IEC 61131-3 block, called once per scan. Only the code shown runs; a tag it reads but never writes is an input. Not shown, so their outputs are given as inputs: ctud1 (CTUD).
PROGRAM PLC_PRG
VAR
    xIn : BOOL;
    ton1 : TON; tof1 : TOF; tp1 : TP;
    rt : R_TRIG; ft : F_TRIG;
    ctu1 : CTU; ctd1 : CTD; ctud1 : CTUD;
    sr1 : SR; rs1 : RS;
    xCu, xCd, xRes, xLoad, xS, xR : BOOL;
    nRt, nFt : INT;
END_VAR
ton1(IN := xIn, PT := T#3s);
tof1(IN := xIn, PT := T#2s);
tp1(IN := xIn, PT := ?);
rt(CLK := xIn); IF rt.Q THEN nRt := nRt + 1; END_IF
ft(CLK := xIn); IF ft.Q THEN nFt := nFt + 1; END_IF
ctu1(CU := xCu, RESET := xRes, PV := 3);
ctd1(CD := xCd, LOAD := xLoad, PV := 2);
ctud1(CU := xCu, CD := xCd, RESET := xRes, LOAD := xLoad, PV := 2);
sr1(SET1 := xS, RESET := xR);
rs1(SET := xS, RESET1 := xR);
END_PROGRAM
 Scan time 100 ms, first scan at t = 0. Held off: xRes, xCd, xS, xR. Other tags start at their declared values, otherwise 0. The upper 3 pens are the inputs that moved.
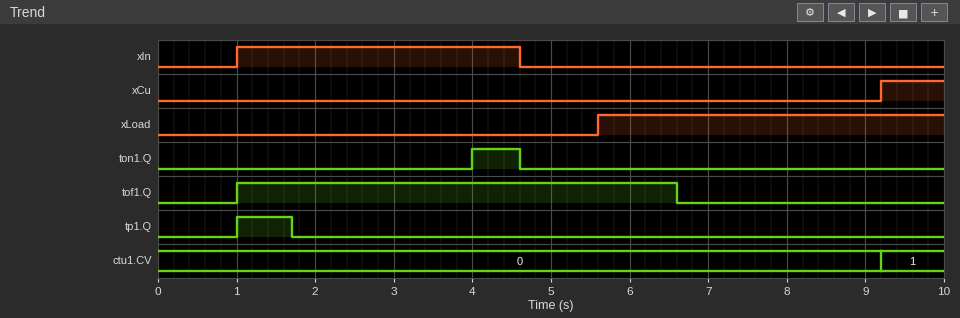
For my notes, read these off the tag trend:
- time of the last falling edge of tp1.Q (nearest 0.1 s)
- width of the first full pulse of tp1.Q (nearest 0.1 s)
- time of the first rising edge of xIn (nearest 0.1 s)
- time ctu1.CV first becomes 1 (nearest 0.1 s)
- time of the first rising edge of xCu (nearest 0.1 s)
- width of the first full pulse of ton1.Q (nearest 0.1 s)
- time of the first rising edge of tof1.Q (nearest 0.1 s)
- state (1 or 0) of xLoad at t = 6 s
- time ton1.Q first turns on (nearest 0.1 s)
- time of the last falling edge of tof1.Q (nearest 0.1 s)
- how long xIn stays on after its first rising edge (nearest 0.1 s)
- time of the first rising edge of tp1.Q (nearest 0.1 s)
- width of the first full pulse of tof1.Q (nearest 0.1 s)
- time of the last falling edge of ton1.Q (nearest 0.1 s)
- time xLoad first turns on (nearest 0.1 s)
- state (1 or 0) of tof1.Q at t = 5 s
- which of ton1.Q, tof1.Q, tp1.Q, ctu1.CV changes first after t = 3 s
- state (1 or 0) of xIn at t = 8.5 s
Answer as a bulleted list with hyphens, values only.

- 1.7 s
- 0.7 s
- 1.0 s
- 9.2 s
- 9.2 s
- 0.6 s
- 1.0 s
- 1
- 4.0 s
- 6.6 s
- 3.6 s
- 1.0 s
- 5.6 s
- 4.6 s
- 5.6 s
- 1
- ton1.Q
- 0
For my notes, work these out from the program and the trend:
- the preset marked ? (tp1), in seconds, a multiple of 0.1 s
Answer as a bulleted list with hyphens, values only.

- 0.7 s
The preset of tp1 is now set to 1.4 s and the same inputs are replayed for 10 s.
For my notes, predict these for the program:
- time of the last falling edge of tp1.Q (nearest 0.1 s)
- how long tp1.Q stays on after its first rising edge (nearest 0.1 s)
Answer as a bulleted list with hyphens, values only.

- 2.4 s
- 1.4 s
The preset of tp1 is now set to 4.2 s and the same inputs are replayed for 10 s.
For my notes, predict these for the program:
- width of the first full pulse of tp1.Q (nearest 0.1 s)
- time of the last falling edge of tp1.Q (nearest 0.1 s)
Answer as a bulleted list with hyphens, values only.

- 4.2 s
- 5.2 s
